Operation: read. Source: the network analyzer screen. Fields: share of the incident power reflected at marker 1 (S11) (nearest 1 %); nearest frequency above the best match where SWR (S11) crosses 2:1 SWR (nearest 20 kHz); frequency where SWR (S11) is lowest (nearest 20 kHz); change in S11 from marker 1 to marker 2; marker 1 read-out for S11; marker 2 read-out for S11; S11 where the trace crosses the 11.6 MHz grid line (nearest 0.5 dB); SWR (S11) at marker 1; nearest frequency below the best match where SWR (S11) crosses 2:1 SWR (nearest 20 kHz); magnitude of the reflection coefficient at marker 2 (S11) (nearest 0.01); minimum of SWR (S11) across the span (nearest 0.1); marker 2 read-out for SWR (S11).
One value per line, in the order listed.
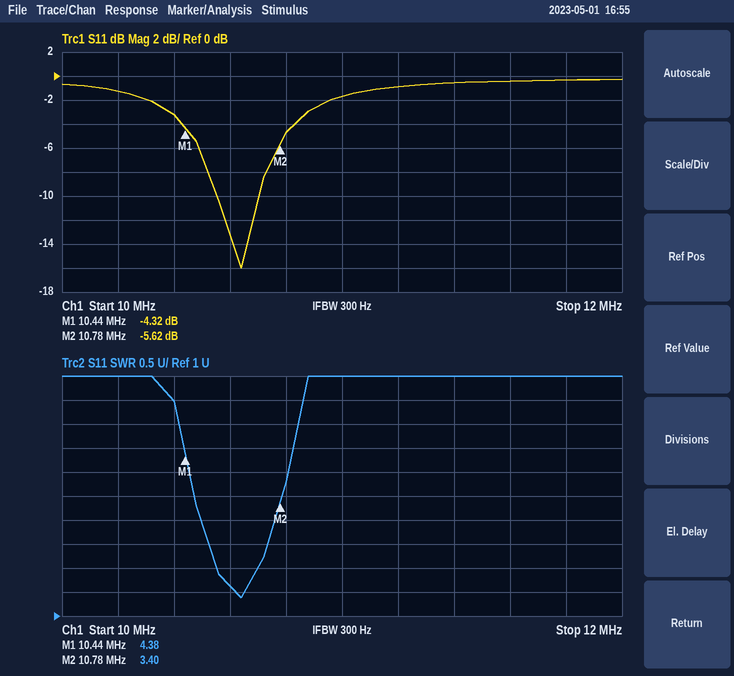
37 %
10.70 MHz
10.64 MHz
-1.30 dB
-4.32 dB
-5.62 dB
-0.5 dB
4.38
10.56 MHz
0.52
1.4
3.40
